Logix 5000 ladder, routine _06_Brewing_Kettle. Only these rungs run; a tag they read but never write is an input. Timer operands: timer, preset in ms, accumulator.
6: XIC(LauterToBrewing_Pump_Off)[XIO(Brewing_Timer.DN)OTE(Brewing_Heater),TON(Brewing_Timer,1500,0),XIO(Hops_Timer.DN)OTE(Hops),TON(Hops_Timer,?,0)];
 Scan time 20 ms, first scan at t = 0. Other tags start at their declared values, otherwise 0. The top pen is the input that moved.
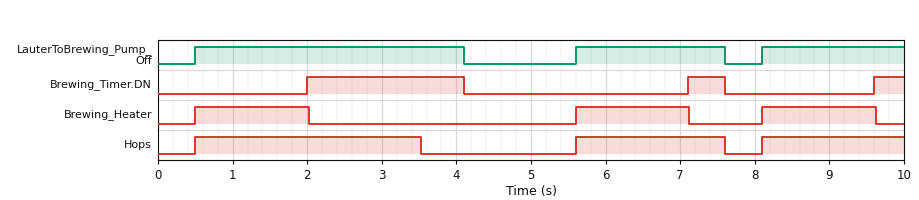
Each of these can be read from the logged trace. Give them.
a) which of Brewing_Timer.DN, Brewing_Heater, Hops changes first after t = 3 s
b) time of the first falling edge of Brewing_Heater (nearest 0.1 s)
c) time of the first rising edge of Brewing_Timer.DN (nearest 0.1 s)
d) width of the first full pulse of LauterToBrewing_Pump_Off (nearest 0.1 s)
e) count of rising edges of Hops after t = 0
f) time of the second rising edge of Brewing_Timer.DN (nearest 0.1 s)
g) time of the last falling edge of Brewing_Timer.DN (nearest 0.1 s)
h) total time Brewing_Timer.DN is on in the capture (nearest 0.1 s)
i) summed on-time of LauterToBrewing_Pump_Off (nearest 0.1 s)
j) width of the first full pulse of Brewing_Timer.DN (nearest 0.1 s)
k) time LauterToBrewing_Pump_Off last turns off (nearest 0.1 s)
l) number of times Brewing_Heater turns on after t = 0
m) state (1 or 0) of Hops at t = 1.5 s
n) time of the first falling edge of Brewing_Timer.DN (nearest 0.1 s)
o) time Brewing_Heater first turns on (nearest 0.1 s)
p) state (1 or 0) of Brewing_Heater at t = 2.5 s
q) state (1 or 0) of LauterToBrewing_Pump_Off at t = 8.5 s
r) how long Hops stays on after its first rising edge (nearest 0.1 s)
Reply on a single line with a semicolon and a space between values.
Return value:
Hops; 2.0 s; 2.0 s; 3.6 s; 3; 7.1 s; 7.6 s; 3.0 s; 7.5 s; 2.1 s; 7.6 s; 3; 1; 4.1 s; 0.5 s; 0; 1; 3.0 s
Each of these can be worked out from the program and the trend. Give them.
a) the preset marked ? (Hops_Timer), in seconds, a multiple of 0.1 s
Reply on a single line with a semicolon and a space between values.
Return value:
3.0 s
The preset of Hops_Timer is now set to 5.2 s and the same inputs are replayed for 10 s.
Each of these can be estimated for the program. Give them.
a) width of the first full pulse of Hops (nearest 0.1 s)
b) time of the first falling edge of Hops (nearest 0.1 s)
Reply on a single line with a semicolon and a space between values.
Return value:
3.6 s; 4.1 s
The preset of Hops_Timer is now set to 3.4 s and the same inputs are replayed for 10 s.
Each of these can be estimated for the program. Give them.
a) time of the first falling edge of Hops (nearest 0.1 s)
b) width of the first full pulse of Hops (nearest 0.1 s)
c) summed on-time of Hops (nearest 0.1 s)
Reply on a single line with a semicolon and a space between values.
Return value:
3.9 s; 3.4 s; 7.3 s
